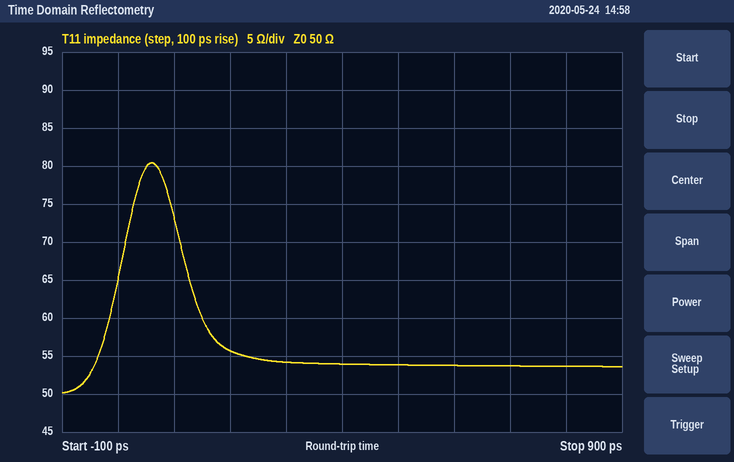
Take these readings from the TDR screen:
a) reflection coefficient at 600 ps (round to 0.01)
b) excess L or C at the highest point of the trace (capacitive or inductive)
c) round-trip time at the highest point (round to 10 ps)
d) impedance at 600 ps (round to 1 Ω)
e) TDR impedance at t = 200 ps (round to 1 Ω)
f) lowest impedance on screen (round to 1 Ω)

+0.04
inductive
60 ps
54 Ω
56 Ω
50 Ω
